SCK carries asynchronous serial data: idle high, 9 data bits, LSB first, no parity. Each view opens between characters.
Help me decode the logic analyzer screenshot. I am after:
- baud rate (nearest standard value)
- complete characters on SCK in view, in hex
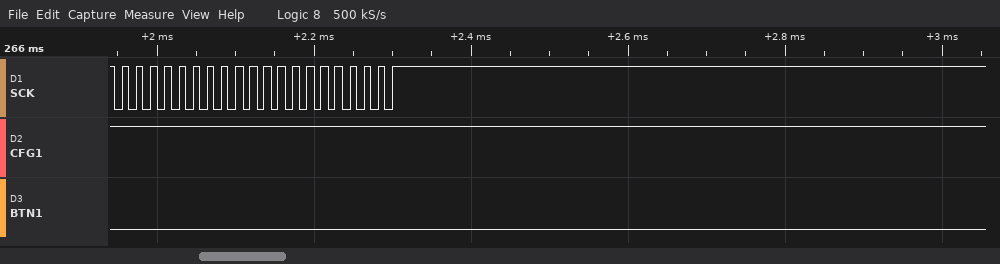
100000 baud
A5, B5, AD, 1FD
